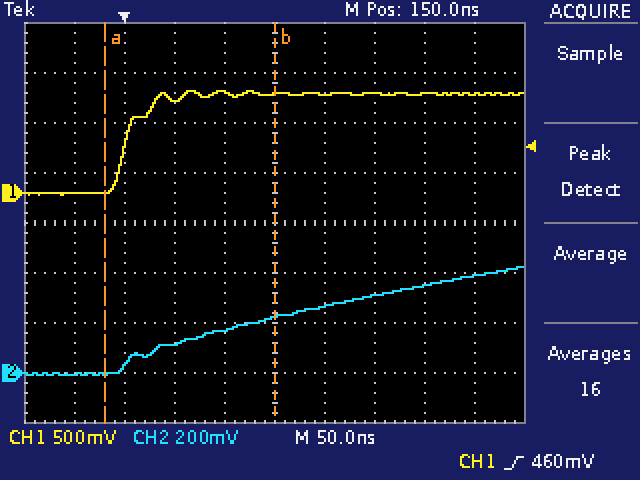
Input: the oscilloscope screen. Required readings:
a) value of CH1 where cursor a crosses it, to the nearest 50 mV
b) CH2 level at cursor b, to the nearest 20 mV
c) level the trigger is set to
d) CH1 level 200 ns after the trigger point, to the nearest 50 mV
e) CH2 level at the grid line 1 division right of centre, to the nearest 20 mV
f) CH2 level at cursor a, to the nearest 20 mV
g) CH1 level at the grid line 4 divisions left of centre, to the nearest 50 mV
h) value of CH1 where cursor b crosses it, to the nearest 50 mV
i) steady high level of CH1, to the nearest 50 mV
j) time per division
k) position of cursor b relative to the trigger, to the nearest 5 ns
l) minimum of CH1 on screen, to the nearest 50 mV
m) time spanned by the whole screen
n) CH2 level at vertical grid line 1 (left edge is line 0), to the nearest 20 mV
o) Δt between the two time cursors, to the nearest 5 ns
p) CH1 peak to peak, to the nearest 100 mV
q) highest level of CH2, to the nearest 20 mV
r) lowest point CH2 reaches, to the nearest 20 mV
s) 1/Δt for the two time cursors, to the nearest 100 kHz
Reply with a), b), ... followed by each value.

a) 0 mV
b) 220 mV
c) 460 mV
d) 1.00 V
e) 260 mV
f) 0 mV
g) 0 mV
h) 1.00 V
i) 1.00 V
j) 50 ns
k) +150 ns
l) 0 mV
m) 500 ns
n) 0 mV
o) 170 ns
p) 1.00 V
q) 420 mV
r) 0 mV
s) 5.9 MHz
